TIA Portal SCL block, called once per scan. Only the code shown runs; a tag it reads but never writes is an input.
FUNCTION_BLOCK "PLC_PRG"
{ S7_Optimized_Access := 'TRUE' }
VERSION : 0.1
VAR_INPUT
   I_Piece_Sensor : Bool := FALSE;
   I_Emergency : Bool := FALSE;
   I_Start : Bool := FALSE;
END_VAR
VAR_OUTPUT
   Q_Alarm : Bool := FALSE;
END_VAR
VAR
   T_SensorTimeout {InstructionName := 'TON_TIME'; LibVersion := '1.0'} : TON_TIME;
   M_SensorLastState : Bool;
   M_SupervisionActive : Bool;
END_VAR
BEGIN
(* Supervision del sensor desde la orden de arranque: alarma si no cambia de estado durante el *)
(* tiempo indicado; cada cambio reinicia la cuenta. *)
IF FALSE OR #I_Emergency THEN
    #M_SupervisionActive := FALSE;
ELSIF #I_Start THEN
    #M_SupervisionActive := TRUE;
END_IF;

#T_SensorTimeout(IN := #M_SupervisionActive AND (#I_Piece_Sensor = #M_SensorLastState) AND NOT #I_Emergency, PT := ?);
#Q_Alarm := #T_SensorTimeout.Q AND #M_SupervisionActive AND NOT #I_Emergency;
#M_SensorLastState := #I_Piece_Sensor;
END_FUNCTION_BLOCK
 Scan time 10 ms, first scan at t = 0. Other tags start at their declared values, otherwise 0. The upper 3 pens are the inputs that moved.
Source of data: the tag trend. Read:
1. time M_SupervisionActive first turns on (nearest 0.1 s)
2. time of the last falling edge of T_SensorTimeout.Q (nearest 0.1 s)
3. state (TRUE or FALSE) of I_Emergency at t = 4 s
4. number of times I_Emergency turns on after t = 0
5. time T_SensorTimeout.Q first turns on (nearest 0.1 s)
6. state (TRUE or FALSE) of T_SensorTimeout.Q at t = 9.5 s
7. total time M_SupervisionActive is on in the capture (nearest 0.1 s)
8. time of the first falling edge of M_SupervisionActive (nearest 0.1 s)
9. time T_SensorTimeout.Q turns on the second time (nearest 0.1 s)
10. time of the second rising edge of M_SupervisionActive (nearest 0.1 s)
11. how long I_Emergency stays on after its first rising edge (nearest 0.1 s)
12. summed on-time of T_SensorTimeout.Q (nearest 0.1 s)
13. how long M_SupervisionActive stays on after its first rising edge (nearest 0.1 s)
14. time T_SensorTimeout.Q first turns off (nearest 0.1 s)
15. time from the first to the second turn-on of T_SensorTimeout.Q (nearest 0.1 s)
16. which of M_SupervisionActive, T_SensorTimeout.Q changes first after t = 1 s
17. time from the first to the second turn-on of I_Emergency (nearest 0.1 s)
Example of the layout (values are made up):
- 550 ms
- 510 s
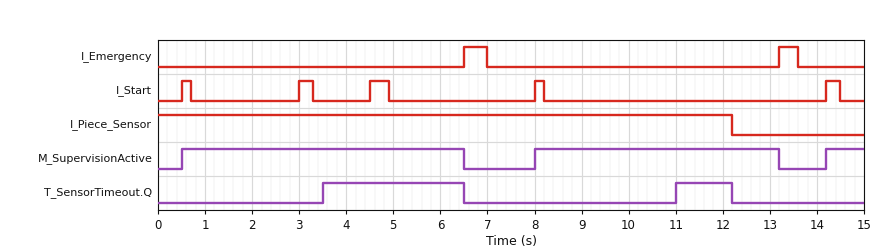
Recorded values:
- 0.5 s
- 12.2 s
- FALSE
- 2
- 3.5 s
- FALSE
- 12.0 s
- 6.5 s
- 11.0 s
- 8.0 s
- 0.5 s
- 4.2 s
- 6.0 s
- 6.5 s
- 7.5 s
- T_SensorTimeout.Q
- 6.7 s
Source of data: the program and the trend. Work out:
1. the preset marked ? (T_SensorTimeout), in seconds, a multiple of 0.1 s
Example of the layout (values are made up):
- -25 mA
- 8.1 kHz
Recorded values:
- 3.0 s
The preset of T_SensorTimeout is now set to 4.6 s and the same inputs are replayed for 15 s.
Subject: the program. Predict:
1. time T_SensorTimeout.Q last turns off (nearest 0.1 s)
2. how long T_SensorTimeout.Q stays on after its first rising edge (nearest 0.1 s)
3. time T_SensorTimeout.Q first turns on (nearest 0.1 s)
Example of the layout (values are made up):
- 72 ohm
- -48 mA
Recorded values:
- 6.5 s
- 1.4 s
- 5.1 s
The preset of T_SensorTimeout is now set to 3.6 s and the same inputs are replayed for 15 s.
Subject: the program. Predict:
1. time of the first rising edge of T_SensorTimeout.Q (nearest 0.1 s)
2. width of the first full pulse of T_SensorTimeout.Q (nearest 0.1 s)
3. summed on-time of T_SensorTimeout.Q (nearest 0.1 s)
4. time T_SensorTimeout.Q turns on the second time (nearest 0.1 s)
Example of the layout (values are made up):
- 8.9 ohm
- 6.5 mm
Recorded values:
- 4.1 s
- 2.4 s
- 3.0 s
- 11.6 s
